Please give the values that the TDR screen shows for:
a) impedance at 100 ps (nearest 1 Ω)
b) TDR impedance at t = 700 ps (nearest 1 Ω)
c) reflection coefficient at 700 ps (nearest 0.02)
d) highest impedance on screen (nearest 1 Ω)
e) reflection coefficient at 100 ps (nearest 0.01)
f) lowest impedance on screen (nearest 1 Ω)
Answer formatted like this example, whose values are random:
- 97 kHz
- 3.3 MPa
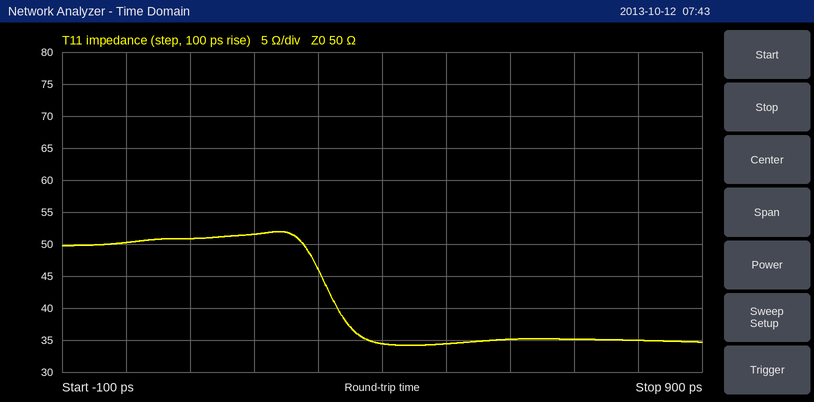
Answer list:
- 51 Ω
- 35 Ω
- -0.18
- 52 Ω
- +0.01
- 34 Ω
